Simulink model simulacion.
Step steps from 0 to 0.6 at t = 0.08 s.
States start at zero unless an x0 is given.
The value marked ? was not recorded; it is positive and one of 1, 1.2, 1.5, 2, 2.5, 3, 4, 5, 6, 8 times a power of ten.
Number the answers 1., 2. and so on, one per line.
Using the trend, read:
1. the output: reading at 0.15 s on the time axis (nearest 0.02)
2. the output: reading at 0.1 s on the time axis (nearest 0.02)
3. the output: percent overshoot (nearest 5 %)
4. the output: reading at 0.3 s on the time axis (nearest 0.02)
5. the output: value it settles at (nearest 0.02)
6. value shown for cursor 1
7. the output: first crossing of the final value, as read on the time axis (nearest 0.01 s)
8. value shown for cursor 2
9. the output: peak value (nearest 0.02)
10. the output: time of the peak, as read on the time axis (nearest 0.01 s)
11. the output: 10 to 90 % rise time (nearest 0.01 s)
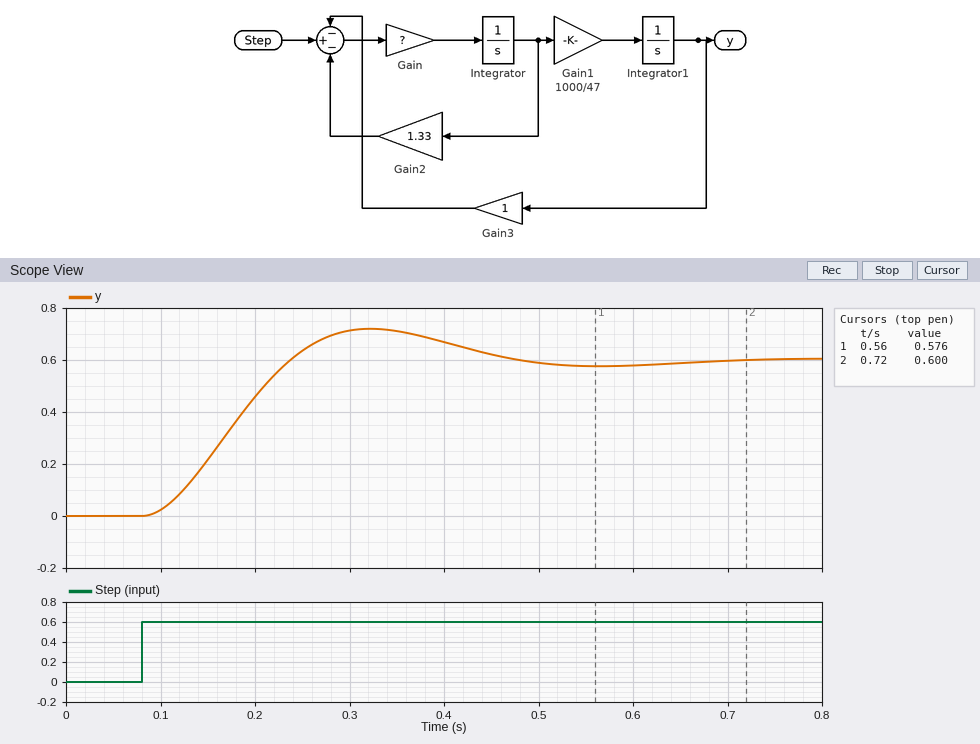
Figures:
1. 0.22
2. 0.02
3. 20 %
4. 0.72
5. 0.60
6. 0.576
7. 0.24 s
8. 0.600
9. 0.72
10. 0.32 s
11. 0.11 s
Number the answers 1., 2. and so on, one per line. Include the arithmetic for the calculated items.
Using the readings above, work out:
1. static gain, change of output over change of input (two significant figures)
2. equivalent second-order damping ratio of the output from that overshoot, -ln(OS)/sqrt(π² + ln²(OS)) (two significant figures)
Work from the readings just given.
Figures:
1. (0.6 - 0) / (0.6 - 0) = 1.0
2. ln(0.2) = -1.609; 1.609 / sqrt(9.870 + 2.590) = 0.46
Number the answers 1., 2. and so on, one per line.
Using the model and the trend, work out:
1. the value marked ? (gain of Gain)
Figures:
1. 10
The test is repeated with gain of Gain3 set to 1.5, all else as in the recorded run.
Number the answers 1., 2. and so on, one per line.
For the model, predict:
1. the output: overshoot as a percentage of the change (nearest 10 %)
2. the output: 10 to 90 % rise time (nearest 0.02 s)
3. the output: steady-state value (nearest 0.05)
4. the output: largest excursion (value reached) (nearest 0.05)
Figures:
1. 30 %
2. 0.08 s
3. 0.40
4. 0.50
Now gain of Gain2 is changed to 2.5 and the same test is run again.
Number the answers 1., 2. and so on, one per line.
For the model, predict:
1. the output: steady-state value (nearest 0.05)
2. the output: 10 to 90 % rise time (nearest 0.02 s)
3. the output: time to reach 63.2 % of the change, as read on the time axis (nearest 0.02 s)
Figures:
1. 0.60
2. 0.18 s
3. 0.22 s
